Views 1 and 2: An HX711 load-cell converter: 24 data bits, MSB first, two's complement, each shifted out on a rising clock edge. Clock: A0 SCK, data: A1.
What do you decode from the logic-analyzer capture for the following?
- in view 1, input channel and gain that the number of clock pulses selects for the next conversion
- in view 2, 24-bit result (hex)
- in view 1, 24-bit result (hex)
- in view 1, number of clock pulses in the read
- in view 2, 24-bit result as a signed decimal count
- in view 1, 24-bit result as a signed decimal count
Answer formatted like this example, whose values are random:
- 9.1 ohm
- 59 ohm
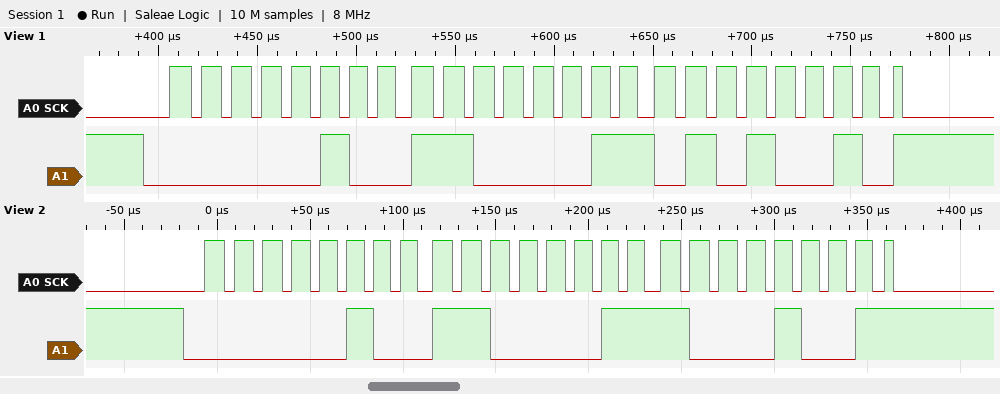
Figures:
- channel A, gain 128
- 0x04C389
- 0x04C352
- 25
- 312201
- 312146
